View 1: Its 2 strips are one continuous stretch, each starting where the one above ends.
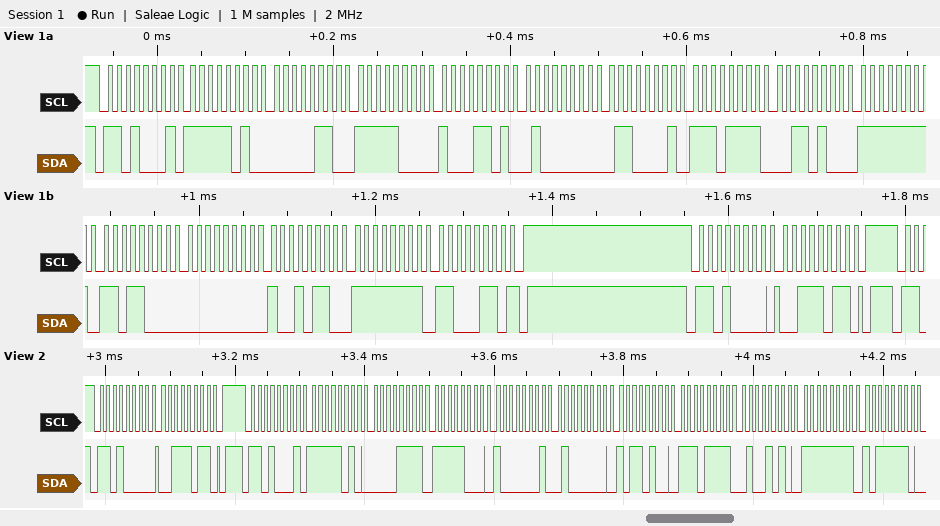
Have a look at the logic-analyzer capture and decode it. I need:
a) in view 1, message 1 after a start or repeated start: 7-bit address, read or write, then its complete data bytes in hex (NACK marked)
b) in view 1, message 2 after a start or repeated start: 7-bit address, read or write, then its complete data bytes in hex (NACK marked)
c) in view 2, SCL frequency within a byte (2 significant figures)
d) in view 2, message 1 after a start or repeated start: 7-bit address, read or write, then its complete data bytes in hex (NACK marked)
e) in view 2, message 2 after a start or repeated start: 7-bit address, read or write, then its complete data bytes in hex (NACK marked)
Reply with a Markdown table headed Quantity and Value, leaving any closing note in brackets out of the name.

| Quantity | Value |
|---|---|
| in view 1, message 1 after a start or repeated start: 7-bit address, read or write, then its complete data bytes in hex | 0x68 read: FA 06 F8 8D 40 61 EF 34 FF D8 00 96 FF C6 NACK |
| in view 1, message 2 after a start or repeated start: 7-bit address, read or write, then its complete data bytes in hex | 0x68 write: 3B |
| in view 2, SCL frequency within a byte | 100 kHz |
| in view 2, message 1 after a start or repeated start: 7-bit address, read or write, then its complete data bytes in hex | 0x68 write: 3B |
| in view 2, message 2 after a start or repeated start: 7-bit address, read or write, then its complete data bytes in hex | 0x68 read: FA 0F F8 81 40 B4 EF 4A FF BE |
